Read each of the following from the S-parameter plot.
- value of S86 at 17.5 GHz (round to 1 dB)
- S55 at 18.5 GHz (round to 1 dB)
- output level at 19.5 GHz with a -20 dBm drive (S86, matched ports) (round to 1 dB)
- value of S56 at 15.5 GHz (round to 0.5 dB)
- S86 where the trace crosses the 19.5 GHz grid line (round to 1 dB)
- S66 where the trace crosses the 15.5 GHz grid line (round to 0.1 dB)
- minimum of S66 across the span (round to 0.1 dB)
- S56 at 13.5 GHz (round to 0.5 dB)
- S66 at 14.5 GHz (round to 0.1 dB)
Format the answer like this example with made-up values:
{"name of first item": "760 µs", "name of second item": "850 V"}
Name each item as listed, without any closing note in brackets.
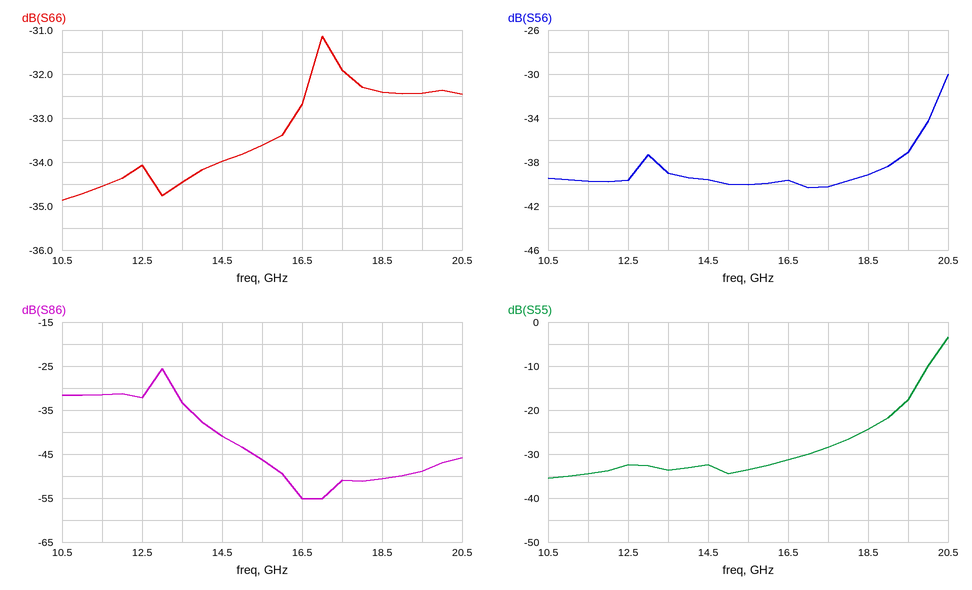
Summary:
{"value of S86 at 17.5 GHz": "-51 dB", "S55 at 18.5 GHz": "-24 dB", "output level at 19.5 GHz with a -20 dBm drive (S86, matched ports)": "-69 dBm", "value of S56 at 15.5 GHz": "-40.0 dB", "S86 where the trace crosses the 19.5 GHz grid line": "-49 dB", "S66 where the trace crosses the 15.5 GHz grid line": "-33.6 dB", "minimum of S66 across the span": "-34.9 dB", "S56 at 13.5 GHz": "-39.0 dB", "S66 at 14.5 GHz": "-34.0 dB"}
